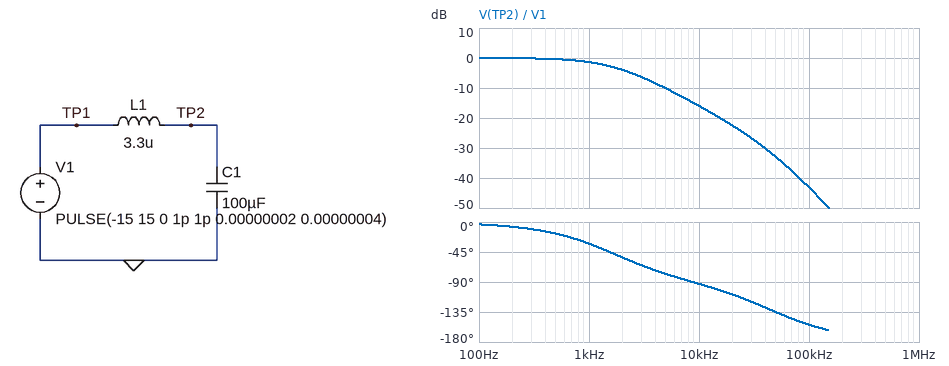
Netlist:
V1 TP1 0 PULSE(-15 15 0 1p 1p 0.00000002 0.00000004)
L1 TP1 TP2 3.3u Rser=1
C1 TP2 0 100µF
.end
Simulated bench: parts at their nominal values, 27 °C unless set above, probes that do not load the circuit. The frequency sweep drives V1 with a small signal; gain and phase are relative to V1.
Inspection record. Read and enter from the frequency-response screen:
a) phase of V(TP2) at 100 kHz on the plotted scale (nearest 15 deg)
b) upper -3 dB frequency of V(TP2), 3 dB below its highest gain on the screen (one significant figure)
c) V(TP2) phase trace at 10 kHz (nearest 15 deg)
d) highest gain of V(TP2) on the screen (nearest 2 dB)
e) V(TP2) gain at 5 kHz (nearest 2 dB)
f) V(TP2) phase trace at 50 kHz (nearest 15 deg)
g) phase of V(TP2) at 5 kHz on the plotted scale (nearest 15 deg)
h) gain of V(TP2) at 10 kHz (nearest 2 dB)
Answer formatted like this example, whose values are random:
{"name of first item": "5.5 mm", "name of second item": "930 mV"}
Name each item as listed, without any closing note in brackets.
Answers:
{"phase of V(TP2) at 100 kHz on the plotted scale": "-150 deg", "upper -3 dB frequency of V(TP2), 3 dB below its highest gain on the screen": "2 kHz", "V(TP2) phase trace at 10 kHz": "-90 deg", "highest gain of V(TP2) on the screen": "0 dB", "V(TP2) gain at 5 kHz": "-10 dB", "V(TP2) phase trace at 50 kHz": "-135 deg", "phase of V(TP2) at 5 kHz on the plotted scale": "-75 deg", "gain of V(TP2) at 10 kHz": "-16 dB"}
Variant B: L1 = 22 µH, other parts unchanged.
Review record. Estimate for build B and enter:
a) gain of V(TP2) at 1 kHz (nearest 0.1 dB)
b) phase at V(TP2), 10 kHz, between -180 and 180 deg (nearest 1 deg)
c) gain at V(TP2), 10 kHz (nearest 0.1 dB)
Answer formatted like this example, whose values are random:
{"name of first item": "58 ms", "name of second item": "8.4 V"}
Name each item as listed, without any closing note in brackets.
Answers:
{"gain of V(TP2) at 1 kHz": "-0.9 dB", "phase at V(TP2), 10 kHz, between -180 and 180 deg": "-141 deg", "gain at V(TP2), 10 kHz": "-19.9 dB"}
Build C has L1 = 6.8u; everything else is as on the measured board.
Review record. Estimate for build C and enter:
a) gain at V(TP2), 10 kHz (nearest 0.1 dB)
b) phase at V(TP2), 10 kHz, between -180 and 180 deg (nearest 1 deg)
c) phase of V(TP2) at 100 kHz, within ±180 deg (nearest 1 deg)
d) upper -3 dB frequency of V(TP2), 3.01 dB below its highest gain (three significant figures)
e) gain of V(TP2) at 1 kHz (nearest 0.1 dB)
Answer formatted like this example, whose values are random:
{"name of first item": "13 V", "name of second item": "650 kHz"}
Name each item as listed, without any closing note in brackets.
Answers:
{"gain at V(TP2), 10 kHz": "-16.3 dB", "phase at V(TP2), 10 kHz, between -180 and 180 deg": "-105 deg", "phase of V(TP2) at 100 kHz, within ±180 deg": "-167 deg", "upper -3 dB frequency of V(TP2), 3.01 dB below its highest gain": "1.71 kHz", "gain of V(TP2) at 1 kHz": "-1.3 dB"}
